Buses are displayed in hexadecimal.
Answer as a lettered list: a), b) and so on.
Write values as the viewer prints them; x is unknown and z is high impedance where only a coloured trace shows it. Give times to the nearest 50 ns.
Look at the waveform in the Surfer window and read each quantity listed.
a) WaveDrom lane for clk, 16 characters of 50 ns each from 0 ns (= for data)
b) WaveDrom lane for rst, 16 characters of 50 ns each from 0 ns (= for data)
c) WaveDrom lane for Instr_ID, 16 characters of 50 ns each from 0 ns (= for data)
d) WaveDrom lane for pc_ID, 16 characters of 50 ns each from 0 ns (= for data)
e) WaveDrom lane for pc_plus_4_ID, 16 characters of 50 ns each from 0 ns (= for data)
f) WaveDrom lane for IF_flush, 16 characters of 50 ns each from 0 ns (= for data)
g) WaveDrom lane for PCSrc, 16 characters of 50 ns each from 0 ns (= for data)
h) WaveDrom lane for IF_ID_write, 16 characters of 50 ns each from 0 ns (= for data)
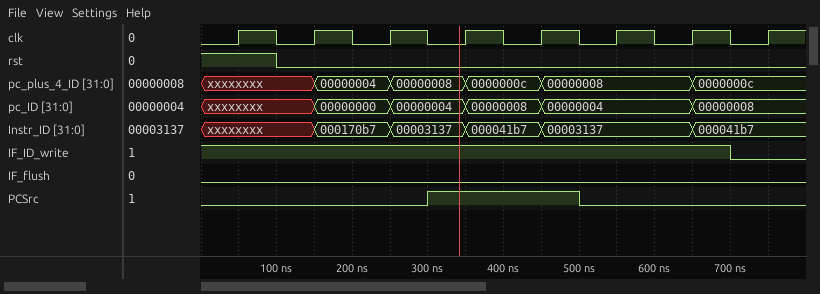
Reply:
a) {name: 'clk', wave: '0101010101010101'}
b) {name: 'rst', wave: '1.0.............'}
c) {name: 'Instr_ID', wave: 'x..=.=.=.=...=..', data: '000170b7 00003137 000041b7 00003137 000041b7'}
d) {name: 'pc_ID', wave: 'x..=.=.=.=...=..', data: '00000000 00000004 00000008 00000004 00000008'}
e) {name: 'pc_plus_4_ID', wave: 'x..=.=.=.=...=..', data: '00000004 00000008 0000000c 00000008 0000000c'}
f) {name: 'IF_flush', wave: '0...............'}
g) {name: 'PCSrc', wave: '0.....1...0.....'}
h) {name: 'IF_ID_write', wave: '1.............0.'}
